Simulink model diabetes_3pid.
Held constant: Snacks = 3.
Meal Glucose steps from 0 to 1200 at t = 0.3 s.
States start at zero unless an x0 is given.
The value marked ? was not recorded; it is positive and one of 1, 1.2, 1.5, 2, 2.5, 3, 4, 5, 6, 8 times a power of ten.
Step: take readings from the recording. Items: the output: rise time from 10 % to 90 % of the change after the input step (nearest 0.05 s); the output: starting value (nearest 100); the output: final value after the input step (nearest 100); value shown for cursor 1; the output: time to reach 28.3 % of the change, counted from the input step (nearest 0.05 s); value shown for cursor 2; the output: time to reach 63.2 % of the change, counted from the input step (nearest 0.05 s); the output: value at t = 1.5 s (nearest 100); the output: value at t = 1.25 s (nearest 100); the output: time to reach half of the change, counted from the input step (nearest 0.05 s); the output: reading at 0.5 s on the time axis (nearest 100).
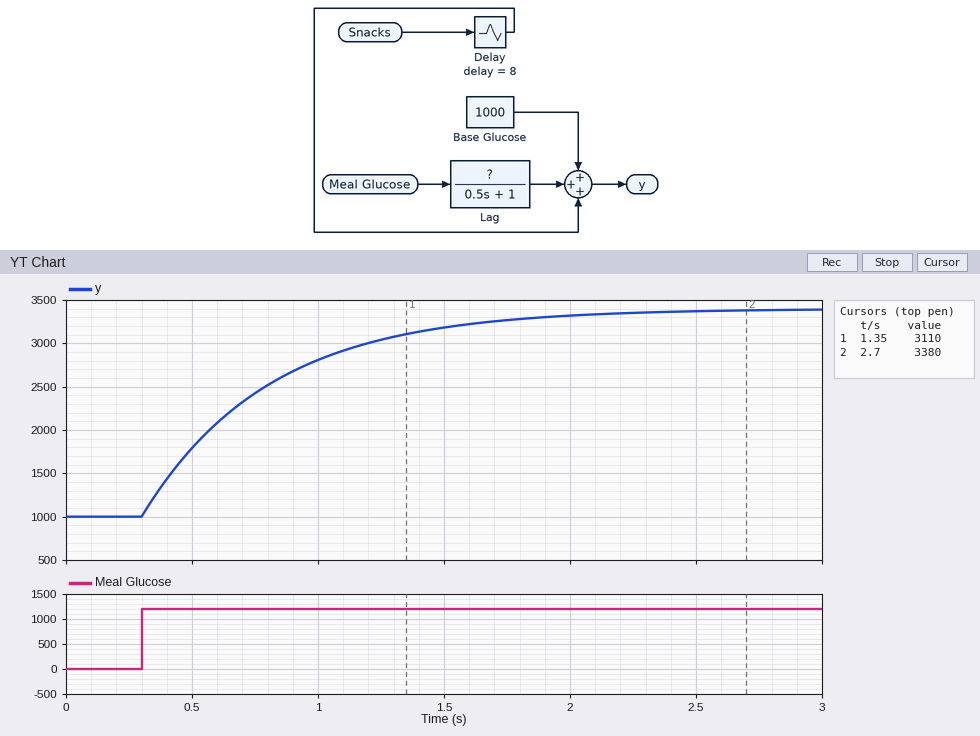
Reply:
1.10 s
1000
3400
3110
0.15 s
3380
0.50 s
3200
3000
0.35 s
1800
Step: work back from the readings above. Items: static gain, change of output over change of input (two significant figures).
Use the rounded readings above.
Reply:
2.0
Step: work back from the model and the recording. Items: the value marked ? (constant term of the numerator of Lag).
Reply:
2
